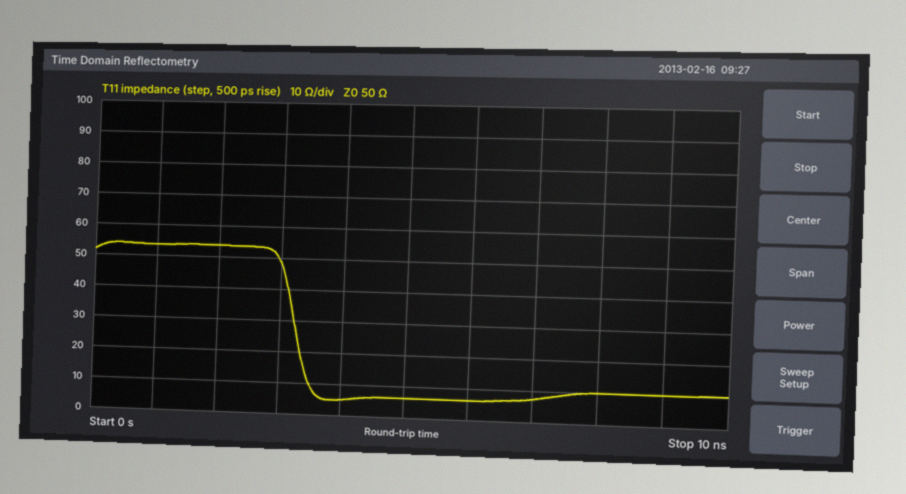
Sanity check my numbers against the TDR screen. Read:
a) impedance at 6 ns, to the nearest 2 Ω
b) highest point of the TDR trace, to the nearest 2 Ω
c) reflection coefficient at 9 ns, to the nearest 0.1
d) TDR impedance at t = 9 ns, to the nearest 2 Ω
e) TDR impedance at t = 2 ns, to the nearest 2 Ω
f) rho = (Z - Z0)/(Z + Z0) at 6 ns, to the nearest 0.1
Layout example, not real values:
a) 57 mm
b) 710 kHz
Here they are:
a) 6 Ω
b) 54 Ω
c) -0.7
d) 10 Ω
e) 54 Ω
f) -0.8
